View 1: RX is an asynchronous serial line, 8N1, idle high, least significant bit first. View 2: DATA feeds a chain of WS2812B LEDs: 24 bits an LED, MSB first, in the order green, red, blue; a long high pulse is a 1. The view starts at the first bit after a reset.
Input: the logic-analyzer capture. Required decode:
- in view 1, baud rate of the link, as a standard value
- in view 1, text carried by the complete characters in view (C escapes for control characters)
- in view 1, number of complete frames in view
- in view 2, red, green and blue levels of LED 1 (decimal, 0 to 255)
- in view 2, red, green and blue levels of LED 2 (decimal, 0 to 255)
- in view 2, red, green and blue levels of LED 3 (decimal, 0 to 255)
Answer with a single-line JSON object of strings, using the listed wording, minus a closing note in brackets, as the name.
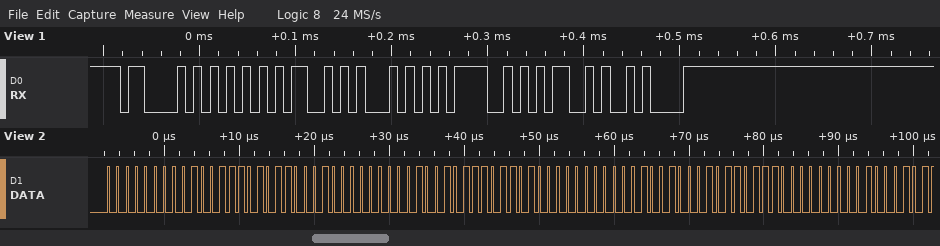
{"in view 1, baud rate of the link, as a standard value": "115200 baud", "in view 1, text carried by the complete characters in view": "\"CUSTOM\\n\"", "in view 1, number of complete frames in view": "7", "in view 2, red, green and blue levels of LED 1": "78, 0, 177", "in view 2, red, green and blue levels of LED 2": "75, 0, 180", "in view 2, red, green and blue levels of LED 3": "72, 0, 183"}
